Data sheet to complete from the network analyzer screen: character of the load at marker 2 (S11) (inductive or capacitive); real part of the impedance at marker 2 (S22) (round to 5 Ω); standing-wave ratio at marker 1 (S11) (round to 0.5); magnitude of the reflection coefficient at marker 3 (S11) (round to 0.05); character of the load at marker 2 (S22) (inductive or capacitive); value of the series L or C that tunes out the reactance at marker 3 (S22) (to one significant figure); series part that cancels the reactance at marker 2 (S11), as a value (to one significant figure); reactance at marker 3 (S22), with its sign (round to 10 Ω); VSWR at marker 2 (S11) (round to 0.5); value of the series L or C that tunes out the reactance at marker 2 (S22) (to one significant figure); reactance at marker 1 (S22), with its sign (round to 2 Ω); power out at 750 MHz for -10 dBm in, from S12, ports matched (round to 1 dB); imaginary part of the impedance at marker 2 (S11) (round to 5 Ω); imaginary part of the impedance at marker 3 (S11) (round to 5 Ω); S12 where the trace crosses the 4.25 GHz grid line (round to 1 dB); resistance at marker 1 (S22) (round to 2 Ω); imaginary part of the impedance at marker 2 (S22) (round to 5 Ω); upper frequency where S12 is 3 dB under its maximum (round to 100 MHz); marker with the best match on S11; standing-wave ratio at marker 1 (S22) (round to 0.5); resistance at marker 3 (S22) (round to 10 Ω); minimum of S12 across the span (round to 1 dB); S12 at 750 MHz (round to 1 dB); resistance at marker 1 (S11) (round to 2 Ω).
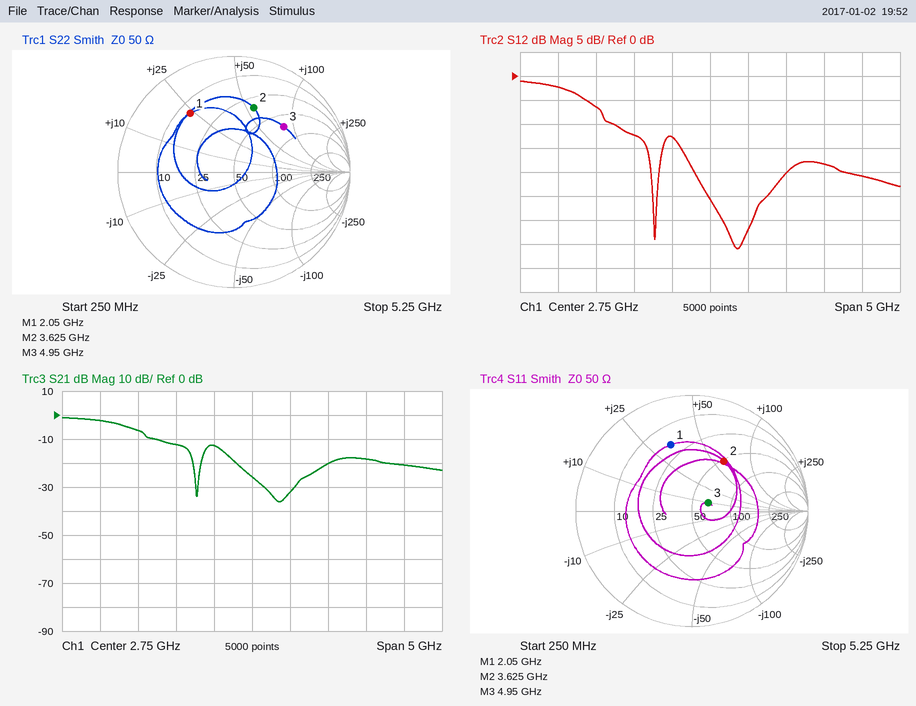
inductive
35 Ω
4.0
0.15
inductive
400 fF
700 fF
+80 Ω
3.0
800 fF
+24 Ω
-12 dBm
+60 Ω
+10 Ω
-18 dB
14 Ω
+55 Ω
1.0 GHz
marker 3
4.5
70 Ω
-36 dB
-2 dB
18 Ω
